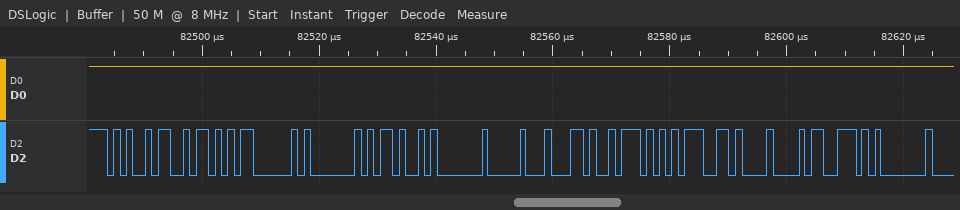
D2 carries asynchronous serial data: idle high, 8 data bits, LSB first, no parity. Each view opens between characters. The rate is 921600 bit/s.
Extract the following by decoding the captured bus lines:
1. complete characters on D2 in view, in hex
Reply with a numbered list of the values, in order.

1. A5, 5A, 03, 01, 2D, 01, 10, 2C, 57, 67, 08, 73, 01
